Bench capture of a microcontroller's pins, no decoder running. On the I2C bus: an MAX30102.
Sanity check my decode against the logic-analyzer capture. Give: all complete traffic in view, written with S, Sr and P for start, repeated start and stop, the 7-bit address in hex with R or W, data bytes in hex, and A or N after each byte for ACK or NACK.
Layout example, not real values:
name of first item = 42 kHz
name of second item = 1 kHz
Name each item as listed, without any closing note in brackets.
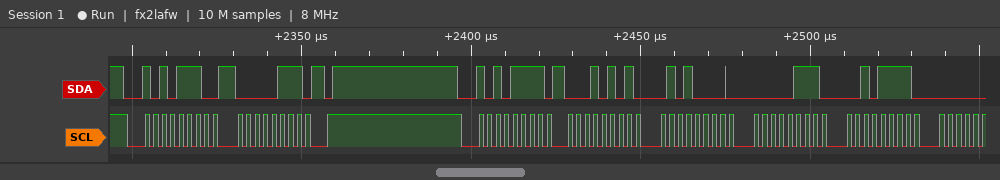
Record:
all complete traffic in view, written with S, Sr and P for start, repeated start and stop, the 7-bit address in hex with R or W, data bytes in hex, and A or N after each byte for ACK or NACK = S 57W A 07 A P S 57R A 15 A 50 A 07 A 2F A
